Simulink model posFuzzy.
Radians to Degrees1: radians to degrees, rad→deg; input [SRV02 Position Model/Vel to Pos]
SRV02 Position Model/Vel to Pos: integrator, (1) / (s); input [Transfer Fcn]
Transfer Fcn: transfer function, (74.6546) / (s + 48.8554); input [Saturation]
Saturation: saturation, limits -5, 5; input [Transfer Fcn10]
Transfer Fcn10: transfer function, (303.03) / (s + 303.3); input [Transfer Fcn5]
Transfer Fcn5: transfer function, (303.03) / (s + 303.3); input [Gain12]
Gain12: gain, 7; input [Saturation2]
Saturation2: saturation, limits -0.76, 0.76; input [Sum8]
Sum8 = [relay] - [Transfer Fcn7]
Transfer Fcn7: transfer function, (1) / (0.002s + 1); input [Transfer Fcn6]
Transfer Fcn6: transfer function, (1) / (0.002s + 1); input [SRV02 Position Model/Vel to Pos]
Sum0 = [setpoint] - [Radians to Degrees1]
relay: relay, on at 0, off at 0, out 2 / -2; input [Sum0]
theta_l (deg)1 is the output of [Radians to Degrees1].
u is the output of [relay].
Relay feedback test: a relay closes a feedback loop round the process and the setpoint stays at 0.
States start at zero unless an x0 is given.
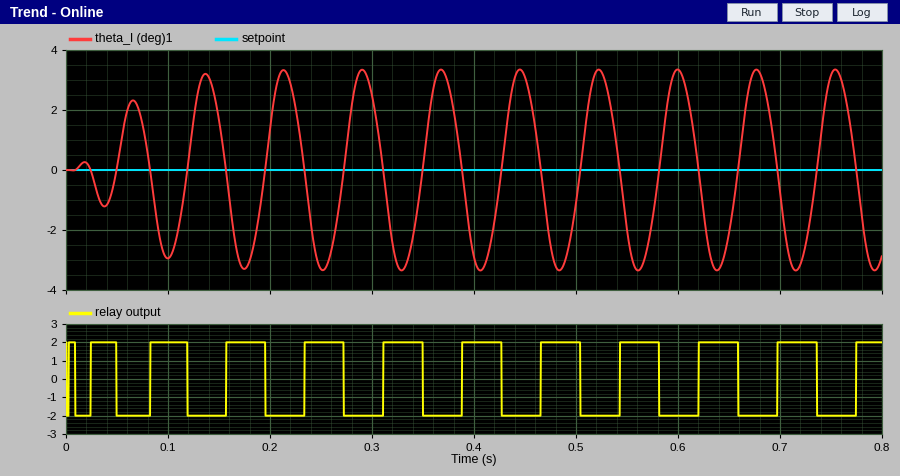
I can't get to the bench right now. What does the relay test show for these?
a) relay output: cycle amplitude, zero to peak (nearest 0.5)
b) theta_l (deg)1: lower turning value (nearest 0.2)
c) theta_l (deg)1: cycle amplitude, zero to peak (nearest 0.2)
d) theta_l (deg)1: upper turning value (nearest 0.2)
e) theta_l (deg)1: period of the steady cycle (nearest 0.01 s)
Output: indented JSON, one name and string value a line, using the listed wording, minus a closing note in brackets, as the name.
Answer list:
{
  "relay output: cycle amplitude, zero to peak": "2.0",
  "theta_l (deg)1: lower turning value": "-3.4",
  "theta_l (deg)1: cycle amplitude, zero to peak": "3.4",
  "theta_l (deg)1: upper turning value": "3.4",
  "theta_l (deg)1: period of the steady cycle": "0.08 s"
}
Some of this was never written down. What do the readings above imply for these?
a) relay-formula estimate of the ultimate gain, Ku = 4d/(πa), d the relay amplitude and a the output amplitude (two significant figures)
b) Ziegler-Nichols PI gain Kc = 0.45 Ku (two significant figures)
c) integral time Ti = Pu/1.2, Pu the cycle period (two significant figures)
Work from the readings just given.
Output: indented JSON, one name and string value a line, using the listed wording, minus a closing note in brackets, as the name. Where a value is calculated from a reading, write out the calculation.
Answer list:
{
  "relay-formula estimate of the ultimate gain, Ku = 4d/(πa), d the relay amplitude and a the output amplitude": "4 × 2 / (π × 3.4) = 0.75",
  "Ziegler-Nichols PI gain Kc = 0.45 Ku": "0.45 × 0.75 = 0.34",
  "integral time Ti = Pu/1.2, Pu the cycle period": "0.08 / 1.2 = 0.067 s"
}
